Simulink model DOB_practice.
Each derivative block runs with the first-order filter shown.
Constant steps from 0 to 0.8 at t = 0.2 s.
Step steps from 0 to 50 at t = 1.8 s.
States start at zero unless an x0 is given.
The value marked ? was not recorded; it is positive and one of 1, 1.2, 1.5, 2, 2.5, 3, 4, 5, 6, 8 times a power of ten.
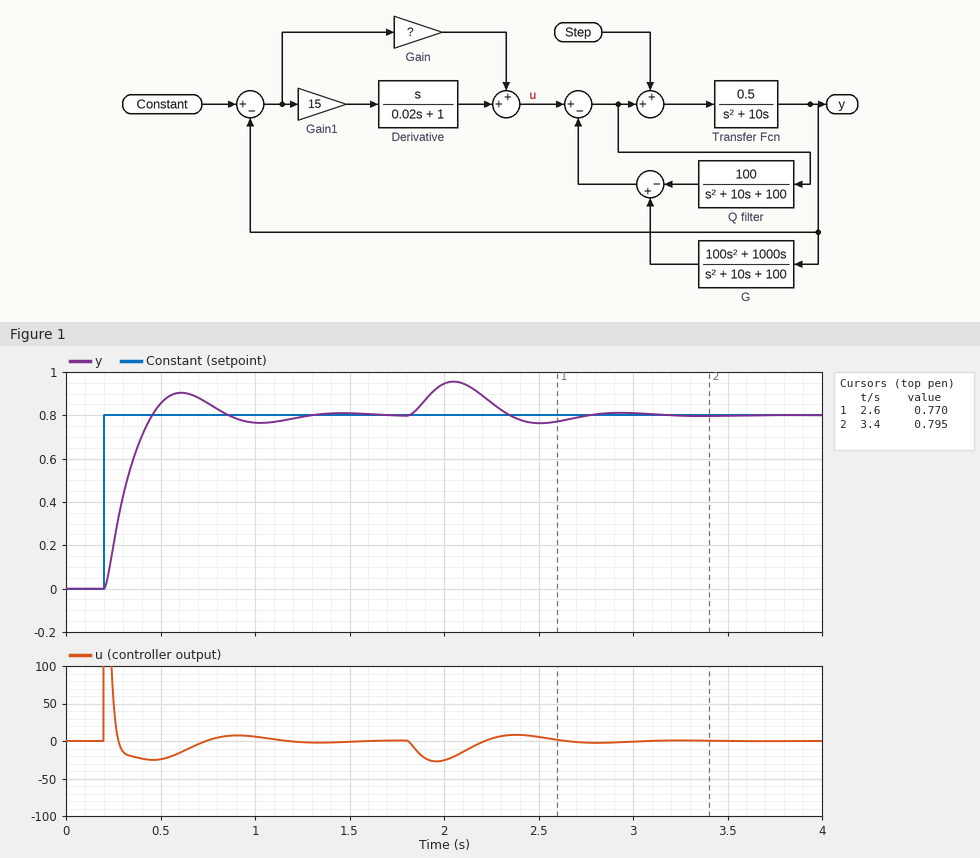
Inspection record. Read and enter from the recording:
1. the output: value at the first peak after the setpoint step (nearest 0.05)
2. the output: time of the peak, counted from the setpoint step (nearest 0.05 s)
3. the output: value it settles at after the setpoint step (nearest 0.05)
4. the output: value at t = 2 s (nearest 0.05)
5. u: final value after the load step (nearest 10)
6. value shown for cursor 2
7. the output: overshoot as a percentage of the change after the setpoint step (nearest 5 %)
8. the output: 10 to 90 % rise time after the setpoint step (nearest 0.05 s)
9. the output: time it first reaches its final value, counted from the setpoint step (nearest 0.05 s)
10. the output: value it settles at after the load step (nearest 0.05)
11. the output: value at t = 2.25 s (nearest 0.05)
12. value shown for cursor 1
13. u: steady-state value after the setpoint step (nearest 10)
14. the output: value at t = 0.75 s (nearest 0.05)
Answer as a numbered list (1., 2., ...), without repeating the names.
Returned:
1. 0.90
2. 0.40 s
3. 0.80
4. 0.95
5. 0
6. 0.795
7. 15 %
8. 0.20 s
9. 0.25 s
10. 0.80
11. 0.85
12. 0.770
13. 0
14. 0.85
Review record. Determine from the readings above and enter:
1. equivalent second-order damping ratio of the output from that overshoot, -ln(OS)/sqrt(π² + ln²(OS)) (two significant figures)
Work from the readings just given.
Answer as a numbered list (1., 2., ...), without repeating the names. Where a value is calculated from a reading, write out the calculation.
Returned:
1. ln(0.15) = -1.897; 1.897 / sqrt(9.870 + 3.599) = 0.52
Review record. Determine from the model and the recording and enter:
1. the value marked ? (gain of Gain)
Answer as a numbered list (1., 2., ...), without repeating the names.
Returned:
1. 120
